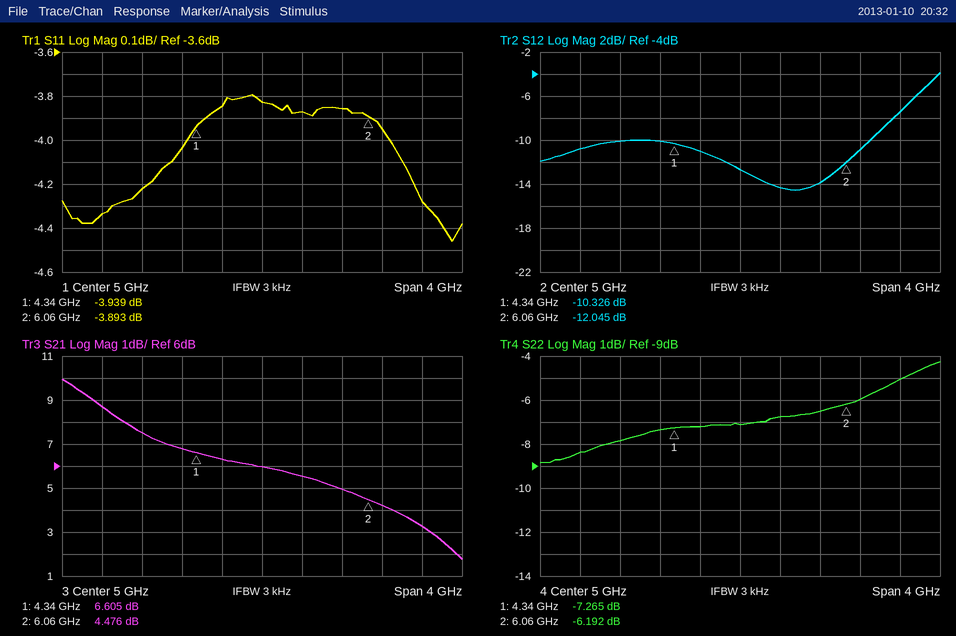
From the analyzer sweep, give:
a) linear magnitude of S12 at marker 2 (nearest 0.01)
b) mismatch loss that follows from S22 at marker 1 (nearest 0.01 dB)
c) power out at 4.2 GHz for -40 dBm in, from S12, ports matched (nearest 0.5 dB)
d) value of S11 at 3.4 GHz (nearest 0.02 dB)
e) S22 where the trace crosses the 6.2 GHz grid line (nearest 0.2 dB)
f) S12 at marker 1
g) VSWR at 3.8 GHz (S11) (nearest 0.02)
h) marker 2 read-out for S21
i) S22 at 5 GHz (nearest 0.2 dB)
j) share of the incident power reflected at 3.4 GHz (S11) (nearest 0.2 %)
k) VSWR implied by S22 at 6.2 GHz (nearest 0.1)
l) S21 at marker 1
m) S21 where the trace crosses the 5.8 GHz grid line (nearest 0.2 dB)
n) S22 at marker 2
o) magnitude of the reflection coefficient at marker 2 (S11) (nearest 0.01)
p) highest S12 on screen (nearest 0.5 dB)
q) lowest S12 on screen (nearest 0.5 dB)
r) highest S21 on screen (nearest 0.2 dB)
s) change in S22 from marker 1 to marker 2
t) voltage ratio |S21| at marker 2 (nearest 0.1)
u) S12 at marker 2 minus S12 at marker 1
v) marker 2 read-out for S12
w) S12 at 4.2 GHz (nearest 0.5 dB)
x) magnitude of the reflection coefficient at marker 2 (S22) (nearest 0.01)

0.25
0.90 dB
-50.0 dBm
-4.34 dB
-6.0 dB
-10.326 dB
4.20
4.476 dB
-7.2 dB
36.8 %
3.0
6.605 dB
5.0 dB
-6.192 dB
0.64
-4.0 dB
-14.5 dB
10.0 dB
1.073 dB
1.7
-1.719 dB
-12.045 dB
-10.0 dB
0.49
